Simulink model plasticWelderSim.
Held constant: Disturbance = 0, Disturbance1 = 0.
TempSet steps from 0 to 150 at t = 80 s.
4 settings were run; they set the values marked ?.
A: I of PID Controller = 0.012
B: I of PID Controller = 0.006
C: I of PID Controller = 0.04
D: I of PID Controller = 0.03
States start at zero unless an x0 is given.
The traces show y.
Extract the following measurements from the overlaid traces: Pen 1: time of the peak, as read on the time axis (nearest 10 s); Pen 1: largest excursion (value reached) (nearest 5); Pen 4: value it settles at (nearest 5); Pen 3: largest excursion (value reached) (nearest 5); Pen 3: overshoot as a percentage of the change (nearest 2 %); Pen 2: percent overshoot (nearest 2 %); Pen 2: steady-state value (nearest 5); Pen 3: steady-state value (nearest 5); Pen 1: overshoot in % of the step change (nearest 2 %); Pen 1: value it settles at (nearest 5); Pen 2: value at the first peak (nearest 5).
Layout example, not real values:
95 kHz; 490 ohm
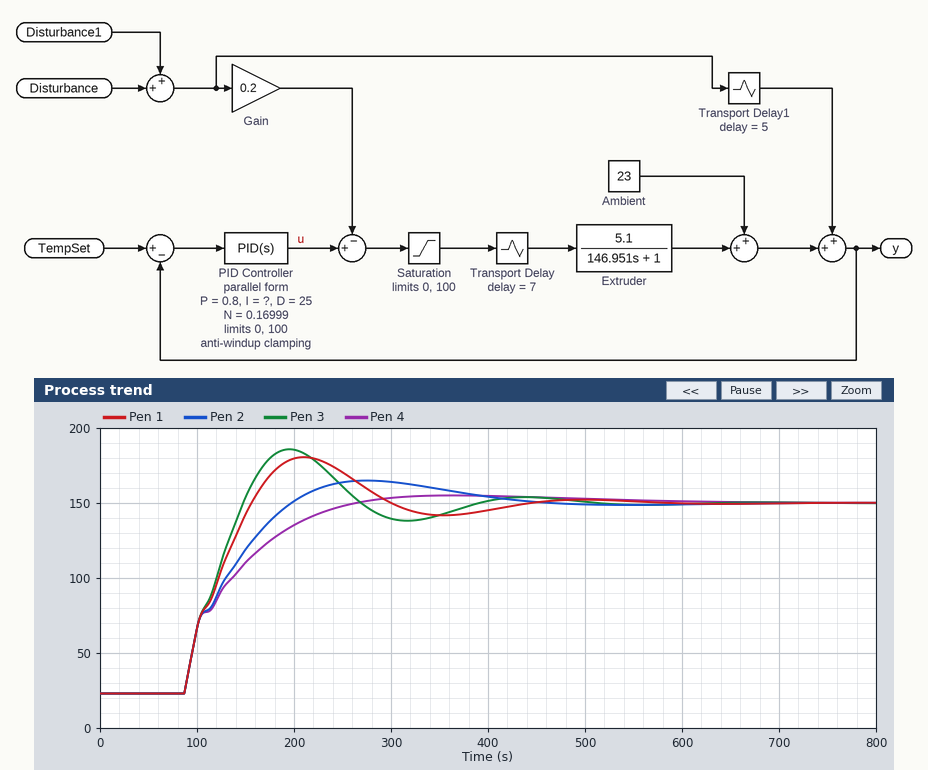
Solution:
210 s; 180; 150; 185; 28 %; 12 %; 150; 150; 24 %; 150; 165
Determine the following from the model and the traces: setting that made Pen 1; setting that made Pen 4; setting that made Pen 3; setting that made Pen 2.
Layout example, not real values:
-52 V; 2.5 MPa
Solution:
D; B; C; A
